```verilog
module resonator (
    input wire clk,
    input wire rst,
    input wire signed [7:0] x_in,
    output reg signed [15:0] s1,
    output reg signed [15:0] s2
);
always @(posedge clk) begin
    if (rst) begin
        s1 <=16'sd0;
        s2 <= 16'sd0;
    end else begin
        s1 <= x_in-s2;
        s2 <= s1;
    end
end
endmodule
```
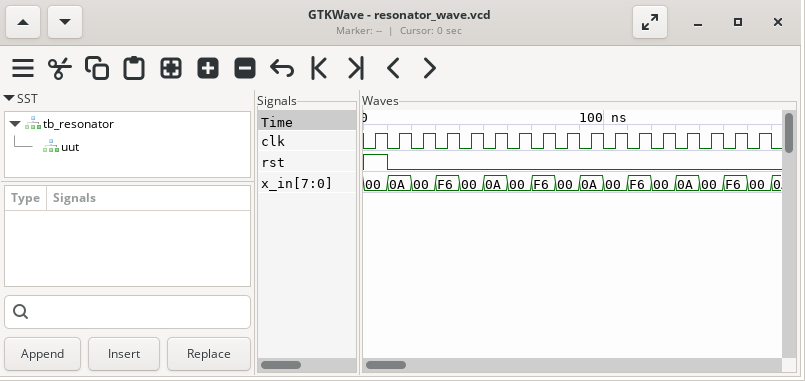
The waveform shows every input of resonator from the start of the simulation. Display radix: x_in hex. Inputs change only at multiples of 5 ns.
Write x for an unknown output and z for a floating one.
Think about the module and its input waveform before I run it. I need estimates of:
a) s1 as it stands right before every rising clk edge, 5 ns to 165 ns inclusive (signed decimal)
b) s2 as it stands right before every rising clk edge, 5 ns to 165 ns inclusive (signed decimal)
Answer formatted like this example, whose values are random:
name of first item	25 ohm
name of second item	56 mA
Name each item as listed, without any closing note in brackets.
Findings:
s1 as it stands right before every rising clk edge, 5 ns to 165 ns inclusive	x, 0, 10, 0, -20, 0, 30, 0, -40, 0, 50, 0, -60, 0, 70, 0, -80
s2 as it stands right before every rising clk edge, 5 ns to 165 ns inclusive	x, 0, 0, 10, 0, -20, 0, 30, 0, -40, 0, 50, 0, -60, 0, 70, 0
